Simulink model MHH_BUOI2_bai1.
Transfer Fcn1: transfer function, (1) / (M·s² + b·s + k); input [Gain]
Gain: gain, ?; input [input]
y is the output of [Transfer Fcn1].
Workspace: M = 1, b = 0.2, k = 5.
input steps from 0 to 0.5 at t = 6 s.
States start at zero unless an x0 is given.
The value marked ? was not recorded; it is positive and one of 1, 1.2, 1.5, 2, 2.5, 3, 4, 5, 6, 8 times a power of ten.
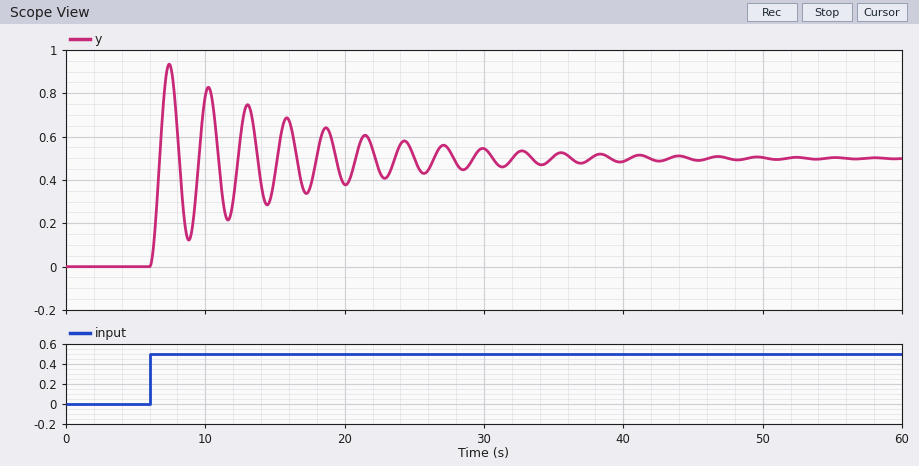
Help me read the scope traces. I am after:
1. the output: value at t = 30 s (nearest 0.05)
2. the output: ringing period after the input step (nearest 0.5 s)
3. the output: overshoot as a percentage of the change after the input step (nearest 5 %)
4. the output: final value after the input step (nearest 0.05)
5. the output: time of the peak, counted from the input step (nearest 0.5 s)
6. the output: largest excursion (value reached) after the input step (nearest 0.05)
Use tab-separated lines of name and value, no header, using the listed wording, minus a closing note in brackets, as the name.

the output: value at t = 30 s	0.55
the output: ringing period after the input step	3.0 s
the output: overshoot as a percentage of the change after the input step	85 %
the output: final value after the input step	0.50
the output: time of the peak, counted from the input step	1.5 s
the output: largest excursion (value reached) after the input step	0.95
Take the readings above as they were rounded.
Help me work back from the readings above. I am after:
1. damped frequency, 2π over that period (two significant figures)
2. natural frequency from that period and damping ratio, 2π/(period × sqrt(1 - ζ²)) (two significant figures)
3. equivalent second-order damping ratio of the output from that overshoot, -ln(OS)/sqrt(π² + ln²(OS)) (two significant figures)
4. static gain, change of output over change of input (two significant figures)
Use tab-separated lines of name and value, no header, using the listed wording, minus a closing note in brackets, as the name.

damped frequency, 2π over that period	2.1 rad/s
natural frequency from that period and damping ratio, 2π/(period × sqrt(1 - ζ²))	2.1 rad/s
equivalent second-order damping ratio of the output from that overshoot, -ln(OS)/sqrt(π² + ln²(OS))	0.052
static gain, change of output over change of input	1.0
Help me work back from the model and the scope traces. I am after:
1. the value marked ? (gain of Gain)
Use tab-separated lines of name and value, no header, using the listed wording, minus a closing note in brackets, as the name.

the value marked ?	5
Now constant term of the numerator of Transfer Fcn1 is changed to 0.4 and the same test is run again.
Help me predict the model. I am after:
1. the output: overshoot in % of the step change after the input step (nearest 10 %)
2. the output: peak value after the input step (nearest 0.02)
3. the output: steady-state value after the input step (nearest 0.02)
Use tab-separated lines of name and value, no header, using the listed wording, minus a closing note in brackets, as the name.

the output: overshoot in % of the step change after the input step	90 %
the output: peak value after the input step	0.38
the output: steady-state value after the input step	0.20
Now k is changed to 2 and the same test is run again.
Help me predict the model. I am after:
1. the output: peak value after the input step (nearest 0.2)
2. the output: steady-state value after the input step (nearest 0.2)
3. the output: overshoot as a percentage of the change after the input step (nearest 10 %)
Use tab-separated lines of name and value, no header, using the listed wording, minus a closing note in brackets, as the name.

the output: peak value after the input step	2.2
the output: steady-state value after the input step	1.2
the output: overshoot as a percentage of the change after the input step	80 %
